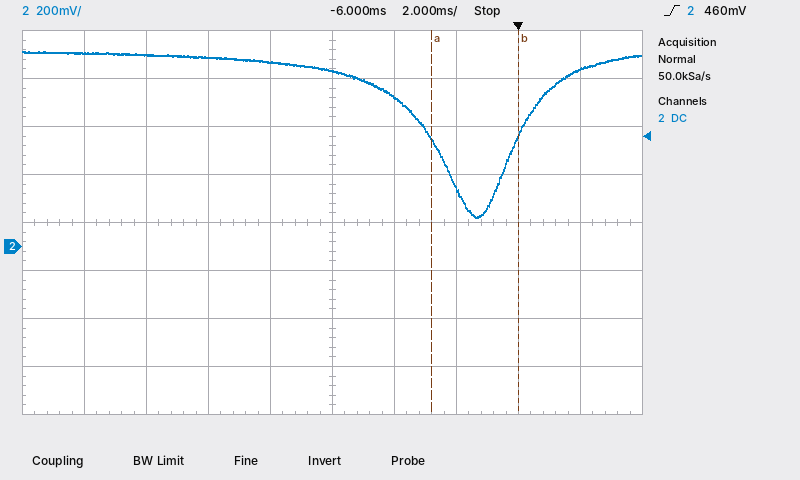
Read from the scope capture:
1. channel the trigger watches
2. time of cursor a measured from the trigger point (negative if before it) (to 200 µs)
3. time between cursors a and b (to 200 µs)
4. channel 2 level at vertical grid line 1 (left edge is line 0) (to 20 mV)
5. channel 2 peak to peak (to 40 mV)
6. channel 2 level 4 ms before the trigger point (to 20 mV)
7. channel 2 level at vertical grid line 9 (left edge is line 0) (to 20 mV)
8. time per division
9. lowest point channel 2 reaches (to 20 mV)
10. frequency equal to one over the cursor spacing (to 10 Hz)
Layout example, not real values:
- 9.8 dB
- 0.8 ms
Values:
- channel 2
- -2.8 ms
- 2.8 ms
- 800 mV
- 680 mV
- 620 mV
- 740 mV
- 2 ms
- 120 mV
- 360 Hz
